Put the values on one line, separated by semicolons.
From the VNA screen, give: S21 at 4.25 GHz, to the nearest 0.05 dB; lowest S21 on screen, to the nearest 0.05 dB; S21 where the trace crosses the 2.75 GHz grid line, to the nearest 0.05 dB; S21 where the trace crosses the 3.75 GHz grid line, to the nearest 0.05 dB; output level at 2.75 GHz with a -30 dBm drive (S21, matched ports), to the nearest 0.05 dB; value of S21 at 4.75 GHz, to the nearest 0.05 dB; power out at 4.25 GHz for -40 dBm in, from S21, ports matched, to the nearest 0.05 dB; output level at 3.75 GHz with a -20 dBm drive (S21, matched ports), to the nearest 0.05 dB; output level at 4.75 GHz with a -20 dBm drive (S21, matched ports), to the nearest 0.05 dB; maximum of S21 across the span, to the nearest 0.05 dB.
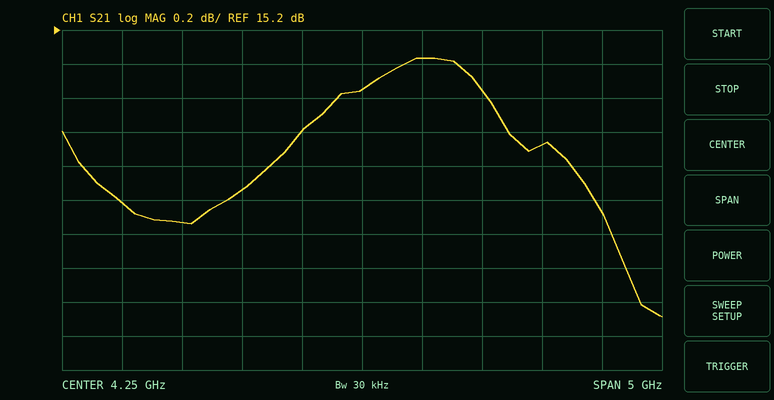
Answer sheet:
14.85 dB; 13.50 dB; 14.05 dB; 14.60 dB; -15.95 dBm; 15.05 dB; -25.15 dBm; -5.40 dBm; -4.95 dBm; 15.05 dB
